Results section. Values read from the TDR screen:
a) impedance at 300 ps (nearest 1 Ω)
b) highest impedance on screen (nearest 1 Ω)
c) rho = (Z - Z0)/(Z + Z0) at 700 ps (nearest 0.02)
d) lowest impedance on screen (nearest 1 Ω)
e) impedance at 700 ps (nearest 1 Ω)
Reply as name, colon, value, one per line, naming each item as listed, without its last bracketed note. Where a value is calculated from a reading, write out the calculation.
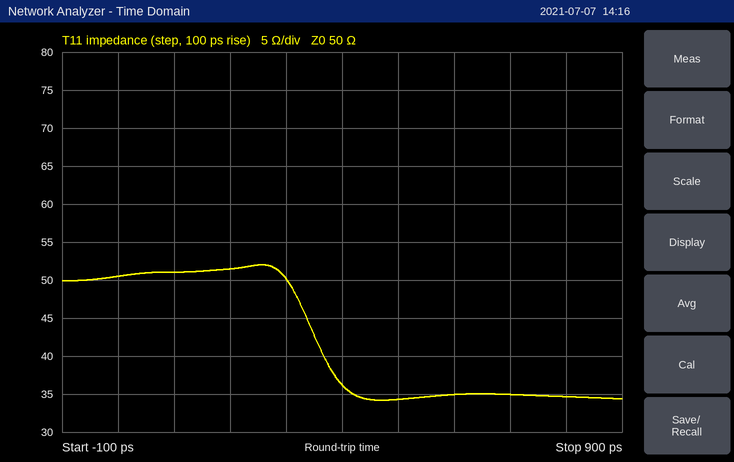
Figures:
impedance at 300 ps: 50 Ω
highest impedance on screen: 52 Ω
rho = (Z - Z0)/(Z + Z0) at 700 ps: (35 − 50)/(35 + 50) ≈ -0.18
lowest impedance on screen: 34 Ω
impedance at 700 ps: 35 Ω
